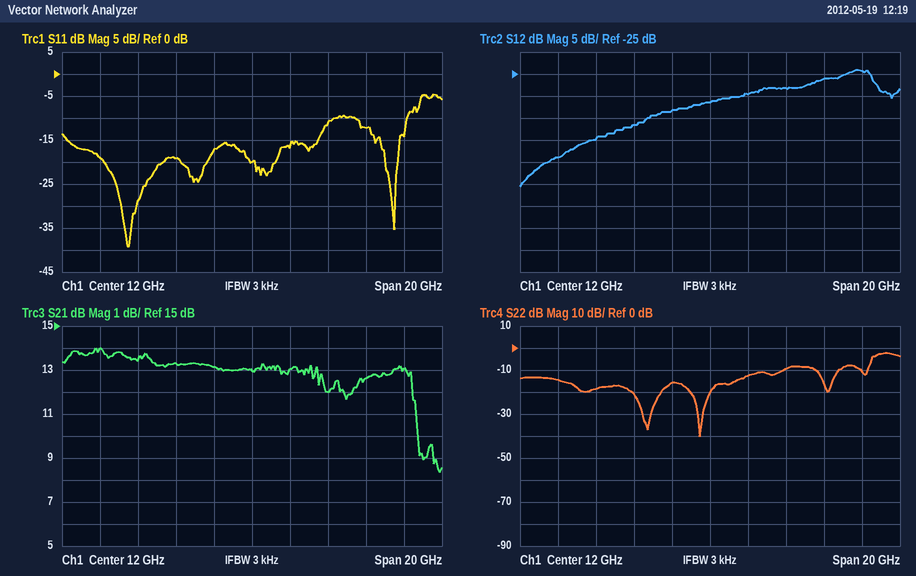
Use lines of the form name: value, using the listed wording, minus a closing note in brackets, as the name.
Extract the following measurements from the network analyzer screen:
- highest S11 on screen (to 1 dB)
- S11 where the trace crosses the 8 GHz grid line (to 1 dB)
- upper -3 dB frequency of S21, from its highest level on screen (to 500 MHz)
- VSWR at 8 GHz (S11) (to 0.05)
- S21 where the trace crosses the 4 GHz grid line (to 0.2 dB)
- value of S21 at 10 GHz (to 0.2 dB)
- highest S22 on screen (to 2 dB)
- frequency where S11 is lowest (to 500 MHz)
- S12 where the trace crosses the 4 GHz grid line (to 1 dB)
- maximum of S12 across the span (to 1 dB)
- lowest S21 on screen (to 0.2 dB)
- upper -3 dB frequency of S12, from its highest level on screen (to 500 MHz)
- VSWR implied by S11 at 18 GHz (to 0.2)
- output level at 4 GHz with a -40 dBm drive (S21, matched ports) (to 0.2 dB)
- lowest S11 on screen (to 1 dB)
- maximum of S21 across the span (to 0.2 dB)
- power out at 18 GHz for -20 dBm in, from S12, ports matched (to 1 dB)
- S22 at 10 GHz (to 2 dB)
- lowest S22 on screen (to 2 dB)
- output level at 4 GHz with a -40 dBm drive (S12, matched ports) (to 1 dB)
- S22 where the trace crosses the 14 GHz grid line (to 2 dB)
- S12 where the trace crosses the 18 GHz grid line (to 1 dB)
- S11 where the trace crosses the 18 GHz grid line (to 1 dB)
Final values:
highest S11 on screen: -5 dB
S11 where the trace crosses the 8 GHz grid line: -19 dB
upper -3 dB frequency of S21, from its highest level on screen: 20.5 GHz
VSWR at 8 GHz (S11): 1.25
S21 where the trace crosses the 4 GHz grid line: 14.0 dB
value of S21 at 10 GHz: 13.2 dB
highest S22 on screen: -2 dB
frequency where S11 is lowest: 5.5 GHz
S12 where the trace crosses the 4 GHz grid line: -44 dB
maximum of S12 across the span: -24 dB
lowest S21 on screen: 8.4 dB
upper -3 dB frequency of S12, from its highest level on screen: 20.5 GHz
VSWR implied by S11 at 18 GHz: 1.6
output level at 4 GHz with a -40 dBm drive (S21, matched ports): -26.0 dBm
lowest S11 on screen: -39 dB
maximum of S21 across the span: 14.0 dB
power out at 18 GHz for -20 dBm in, from S12, ports matched: -46 dBm
S22 at 10 GHz: -16 dB
lowest S22 on screen: -40 dB
output level at 4 GHz with a -40 dBm drive (S12, matched ports): -84 dBm
S22 where the trace crosses the 14 GHz grid line: -12 dB
S12 where the trace crosses the 18 GHz grid line: -26 dB
S11 where the trace crosses the 18 GHz grid line: -12 dB
